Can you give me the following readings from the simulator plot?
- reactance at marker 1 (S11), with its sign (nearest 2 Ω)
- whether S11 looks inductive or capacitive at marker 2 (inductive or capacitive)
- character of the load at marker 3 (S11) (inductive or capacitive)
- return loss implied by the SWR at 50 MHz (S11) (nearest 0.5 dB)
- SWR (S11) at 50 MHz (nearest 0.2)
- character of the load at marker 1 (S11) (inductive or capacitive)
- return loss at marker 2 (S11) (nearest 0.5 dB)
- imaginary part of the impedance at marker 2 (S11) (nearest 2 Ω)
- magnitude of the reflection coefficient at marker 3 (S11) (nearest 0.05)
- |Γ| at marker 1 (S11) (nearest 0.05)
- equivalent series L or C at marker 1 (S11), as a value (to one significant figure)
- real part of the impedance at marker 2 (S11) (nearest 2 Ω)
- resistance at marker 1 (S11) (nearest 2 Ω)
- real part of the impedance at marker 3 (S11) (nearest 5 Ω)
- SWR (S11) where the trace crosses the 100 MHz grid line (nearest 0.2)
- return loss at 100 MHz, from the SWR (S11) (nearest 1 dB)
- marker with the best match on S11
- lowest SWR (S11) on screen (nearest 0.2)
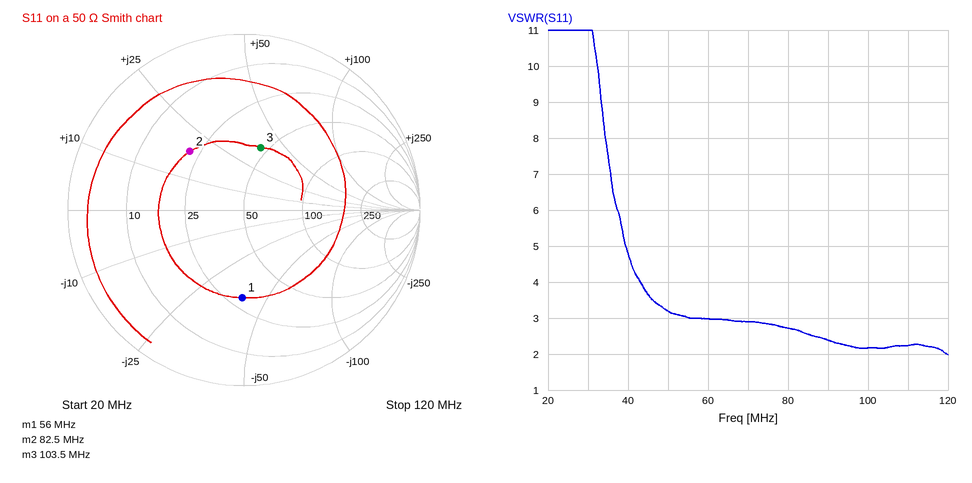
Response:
-40 Ω
inductive
inductive
5.5 dB
3.2
capacitive
7.0 dB
+18 Ω
0.35
0.50
70 pF
22 Ω
30 Ω
45 Ω
2.2
9 dB
marker 3
2.0
